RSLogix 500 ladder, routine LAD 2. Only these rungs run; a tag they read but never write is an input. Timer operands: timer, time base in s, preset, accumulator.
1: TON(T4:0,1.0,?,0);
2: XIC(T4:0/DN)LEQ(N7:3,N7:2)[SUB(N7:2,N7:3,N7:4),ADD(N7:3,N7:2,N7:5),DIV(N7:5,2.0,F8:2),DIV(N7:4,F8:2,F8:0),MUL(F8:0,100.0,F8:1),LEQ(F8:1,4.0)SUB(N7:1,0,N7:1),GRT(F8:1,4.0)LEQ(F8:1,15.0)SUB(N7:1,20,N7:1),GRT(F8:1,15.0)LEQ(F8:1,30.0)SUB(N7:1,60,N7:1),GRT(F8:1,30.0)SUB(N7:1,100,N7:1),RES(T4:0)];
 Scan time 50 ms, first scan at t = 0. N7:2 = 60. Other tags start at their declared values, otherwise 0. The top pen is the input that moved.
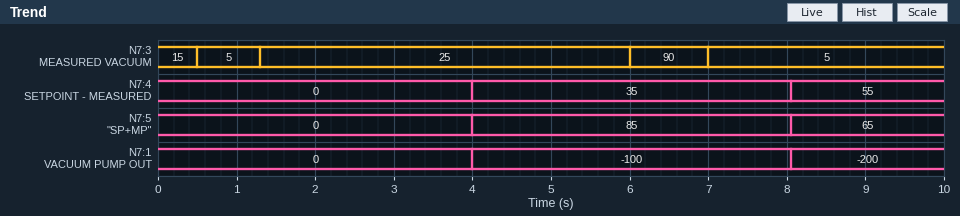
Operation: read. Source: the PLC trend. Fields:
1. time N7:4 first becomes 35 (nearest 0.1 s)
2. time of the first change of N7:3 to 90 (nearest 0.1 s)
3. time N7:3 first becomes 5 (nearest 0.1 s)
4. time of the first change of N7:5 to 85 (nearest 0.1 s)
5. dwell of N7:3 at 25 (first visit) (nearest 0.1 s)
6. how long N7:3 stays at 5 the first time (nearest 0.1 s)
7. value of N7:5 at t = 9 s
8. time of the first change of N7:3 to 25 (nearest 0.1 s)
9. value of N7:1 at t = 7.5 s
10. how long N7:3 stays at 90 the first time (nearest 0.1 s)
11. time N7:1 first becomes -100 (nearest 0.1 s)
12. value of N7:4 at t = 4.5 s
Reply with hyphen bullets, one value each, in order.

- 4.0 s
- 6.0 s
- 0.5 s
- 4.0 s
- 4.7 s
- 0.8 s
- 65
- 1.3 s
- -100
- 1.0 s
- 4.0 s
- 35
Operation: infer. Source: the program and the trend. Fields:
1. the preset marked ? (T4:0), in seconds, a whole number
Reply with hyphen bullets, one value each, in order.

- 4 s
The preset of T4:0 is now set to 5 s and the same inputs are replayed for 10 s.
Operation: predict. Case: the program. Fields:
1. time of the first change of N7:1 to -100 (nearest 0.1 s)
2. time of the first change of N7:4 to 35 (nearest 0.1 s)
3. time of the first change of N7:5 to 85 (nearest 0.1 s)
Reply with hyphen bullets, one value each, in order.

- 5.0 s
- 5.0 s
- 5.0 s
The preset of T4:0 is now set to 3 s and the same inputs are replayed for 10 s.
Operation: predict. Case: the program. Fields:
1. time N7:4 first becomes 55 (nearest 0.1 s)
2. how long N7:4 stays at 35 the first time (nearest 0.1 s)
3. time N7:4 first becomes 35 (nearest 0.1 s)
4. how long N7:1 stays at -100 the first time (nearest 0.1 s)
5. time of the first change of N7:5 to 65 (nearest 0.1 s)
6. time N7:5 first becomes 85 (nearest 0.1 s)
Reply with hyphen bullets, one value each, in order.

- 7.0 s
- 4.0 s
- 3.0 s
- 4.0 s
- 7.0 s
- 3.0 s
